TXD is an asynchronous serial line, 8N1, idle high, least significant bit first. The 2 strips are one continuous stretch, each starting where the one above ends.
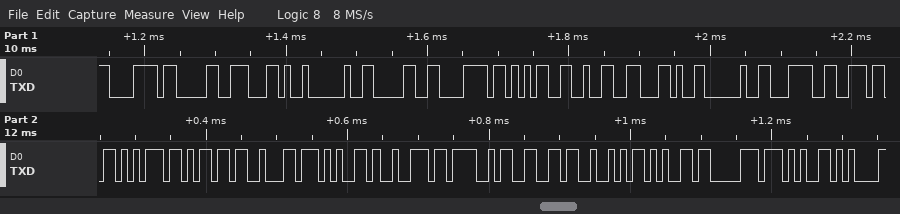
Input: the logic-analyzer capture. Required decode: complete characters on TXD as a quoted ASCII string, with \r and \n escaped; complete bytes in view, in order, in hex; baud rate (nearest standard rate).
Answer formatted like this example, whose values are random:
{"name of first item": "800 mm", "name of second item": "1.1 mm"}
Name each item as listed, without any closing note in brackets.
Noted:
{"complete characters on TXD as a quoted ASCII string, with \\r and \\n escaped": "\"x0, 0x52, <numberOfRepe\"", "complete bytes in view, in order, in hex": "78 30 2C 20 30 78 35 32 2C 20 3C 6E 75 6D 62 65 72 4F 66 52 65 70 65", "baud rate": "115200 baud"}
